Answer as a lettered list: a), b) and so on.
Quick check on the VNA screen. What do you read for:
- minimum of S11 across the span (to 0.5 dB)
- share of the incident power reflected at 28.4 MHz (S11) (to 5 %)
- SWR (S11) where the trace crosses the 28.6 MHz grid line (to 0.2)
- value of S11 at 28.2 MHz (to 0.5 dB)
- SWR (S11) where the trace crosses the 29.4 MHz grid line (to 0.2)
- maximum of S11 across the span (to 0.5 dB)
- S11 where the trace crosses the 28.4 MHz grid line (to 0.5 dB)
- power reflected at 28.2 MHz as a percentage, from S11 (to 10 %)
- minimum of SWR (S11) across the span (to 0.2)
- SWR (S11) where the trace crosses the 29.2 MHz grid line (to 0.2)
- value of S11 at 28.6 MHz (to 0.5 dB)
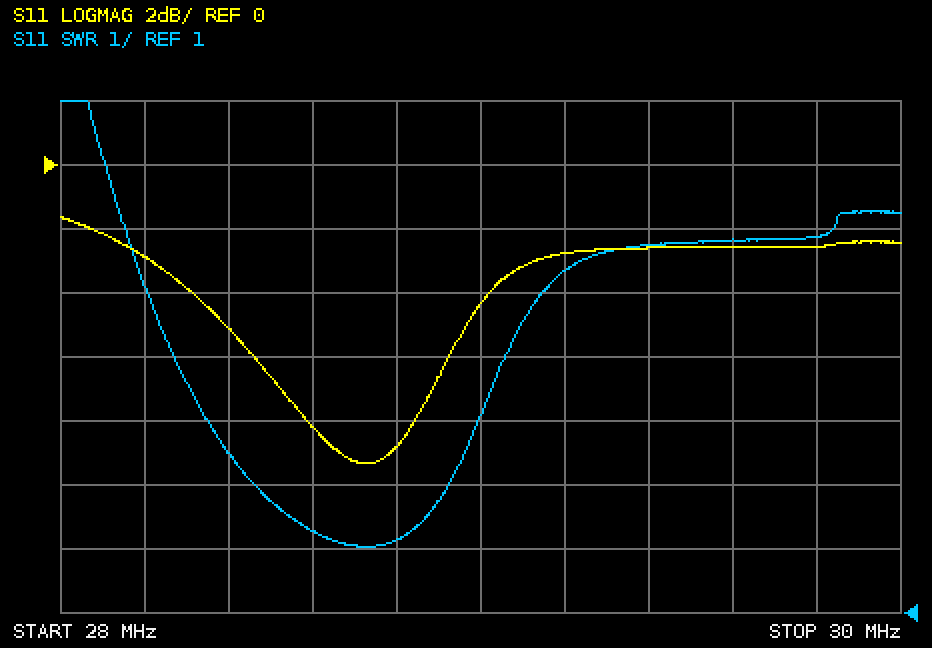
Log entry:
a) -9.5 dB
b) 30 %
c) 2.2
d) -3.0 dB
e) 6.8
f) -1.5 dB
g) -5.0 dB
h) 50 %
i) 2.0
j) 6.4
k) -8.0 dB
